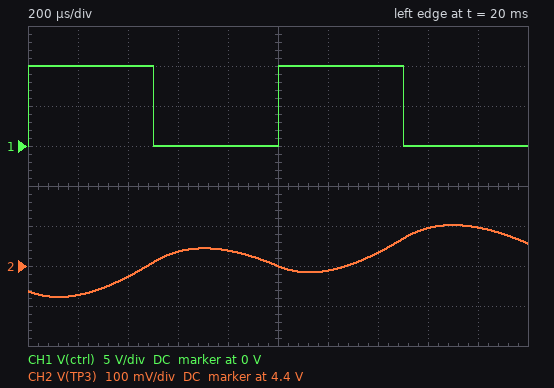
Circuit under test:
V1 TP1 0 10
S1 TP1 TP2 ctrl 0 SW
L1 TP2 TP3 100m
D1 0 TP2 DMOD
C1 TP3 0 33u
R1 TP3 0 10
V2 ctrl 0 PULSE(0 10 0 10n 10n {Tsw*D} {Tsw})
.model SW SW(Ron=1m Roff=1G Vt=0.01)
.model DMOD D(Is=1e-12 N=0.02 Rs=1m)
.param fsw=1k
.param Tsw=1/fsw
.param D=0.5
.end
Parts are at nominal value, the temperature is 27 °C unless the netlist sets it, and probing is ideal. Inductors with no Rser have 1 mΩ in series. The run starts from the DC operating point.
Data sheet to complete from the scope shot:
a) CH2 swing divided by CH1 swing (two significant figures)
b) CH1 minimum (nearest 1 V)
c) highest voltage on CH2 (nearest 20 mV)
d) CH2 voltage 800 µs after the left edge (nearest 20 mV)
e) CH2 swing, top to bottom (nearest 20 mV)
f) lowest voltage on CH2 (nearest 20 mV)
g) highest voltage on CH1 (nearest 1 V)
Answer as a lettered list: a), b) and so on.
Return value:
a) 0.018
b) 0 V
c) 4.50 V
d) 4.44 V
e) 180 mV
f) 4.32 V
g) 10 V
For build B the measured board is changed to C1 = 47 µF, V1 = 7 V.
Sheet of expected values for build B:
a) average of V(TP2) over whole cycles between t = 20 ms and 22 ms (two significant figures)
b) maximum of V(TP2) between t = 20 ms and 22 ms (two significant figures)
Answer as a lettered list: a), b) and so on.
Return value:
a) 3.5 V
b) 7.0 V
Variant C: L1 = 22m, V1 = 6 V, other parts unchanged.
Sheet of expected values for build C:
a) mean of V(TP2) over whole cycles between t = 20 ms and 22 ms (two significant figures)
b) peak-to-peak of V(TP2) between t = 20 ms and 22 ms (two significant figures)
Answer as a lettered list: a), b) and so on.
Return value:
a) 3.0 V
b) 6.0 V
